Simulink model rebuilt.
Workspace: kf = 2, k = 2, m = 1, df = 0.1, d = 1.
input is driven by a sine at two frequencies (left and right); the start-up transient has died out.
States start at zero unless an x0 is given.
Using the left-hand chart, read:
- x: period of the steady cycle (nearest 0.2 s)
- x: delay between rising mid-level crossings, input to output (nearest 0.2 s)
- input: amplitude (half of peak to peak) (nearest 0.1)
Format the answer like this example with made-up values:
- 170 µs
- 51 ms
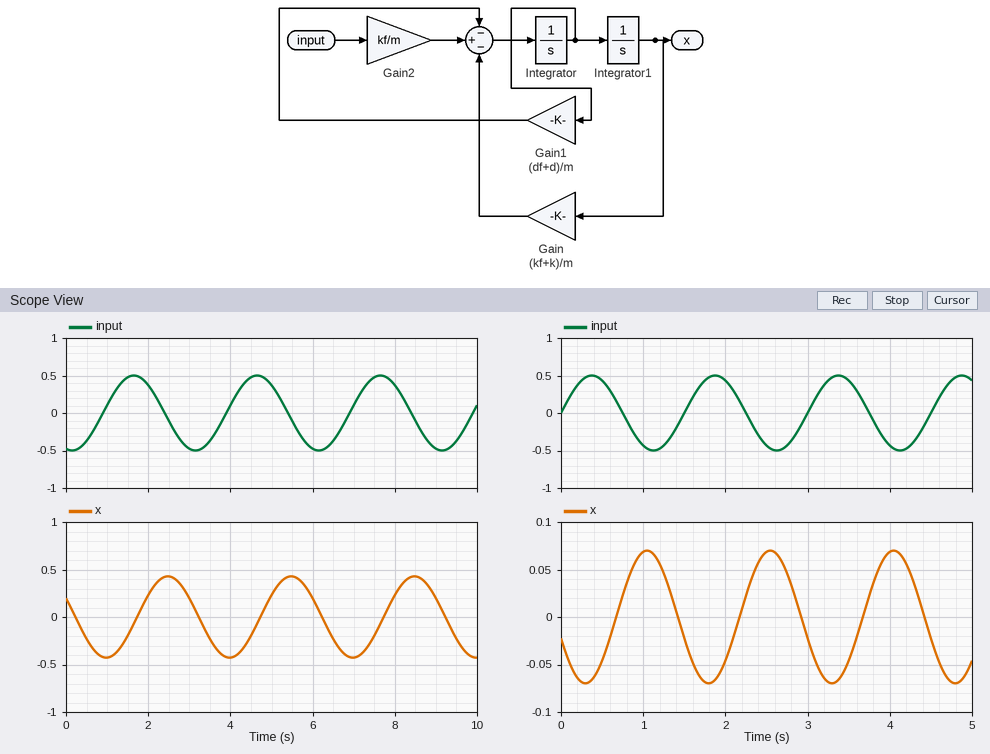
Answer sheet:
- 3.0 s
- 0.8 s
- 0.5
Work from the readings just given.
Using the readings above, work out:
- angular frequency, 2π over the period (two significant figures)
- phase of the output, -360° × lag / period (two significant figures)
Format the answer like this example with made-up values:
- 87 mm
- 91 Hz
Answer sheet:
- 2.1 rad/s
- -96°
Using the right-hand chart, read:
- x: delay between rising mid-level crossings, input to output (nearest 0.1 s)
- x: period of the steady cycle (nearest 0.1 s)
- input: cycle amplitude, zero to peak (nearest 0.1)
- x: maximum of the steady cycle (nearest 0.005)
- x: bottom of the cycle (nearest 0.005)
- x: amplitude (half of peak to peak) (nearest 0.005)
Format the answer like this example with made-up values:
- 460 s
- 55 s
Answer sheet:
- 0.7 s
- 1.5 s
- 0.5
- 0.070
- -0.070
- 0.070
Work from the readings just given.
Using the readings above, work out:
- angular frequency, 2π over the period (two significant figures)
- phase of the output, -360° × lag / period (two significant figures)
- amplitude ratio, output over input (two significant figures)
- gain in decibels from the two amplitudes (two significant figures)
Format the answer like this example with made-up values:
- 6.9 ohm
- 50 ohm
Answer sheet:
- 4.2 rad/s
- -170°
- 0.14
- -17 dB
